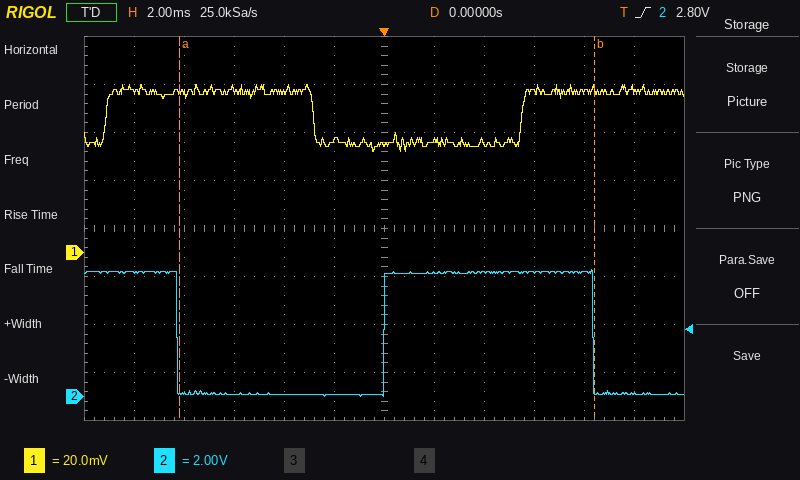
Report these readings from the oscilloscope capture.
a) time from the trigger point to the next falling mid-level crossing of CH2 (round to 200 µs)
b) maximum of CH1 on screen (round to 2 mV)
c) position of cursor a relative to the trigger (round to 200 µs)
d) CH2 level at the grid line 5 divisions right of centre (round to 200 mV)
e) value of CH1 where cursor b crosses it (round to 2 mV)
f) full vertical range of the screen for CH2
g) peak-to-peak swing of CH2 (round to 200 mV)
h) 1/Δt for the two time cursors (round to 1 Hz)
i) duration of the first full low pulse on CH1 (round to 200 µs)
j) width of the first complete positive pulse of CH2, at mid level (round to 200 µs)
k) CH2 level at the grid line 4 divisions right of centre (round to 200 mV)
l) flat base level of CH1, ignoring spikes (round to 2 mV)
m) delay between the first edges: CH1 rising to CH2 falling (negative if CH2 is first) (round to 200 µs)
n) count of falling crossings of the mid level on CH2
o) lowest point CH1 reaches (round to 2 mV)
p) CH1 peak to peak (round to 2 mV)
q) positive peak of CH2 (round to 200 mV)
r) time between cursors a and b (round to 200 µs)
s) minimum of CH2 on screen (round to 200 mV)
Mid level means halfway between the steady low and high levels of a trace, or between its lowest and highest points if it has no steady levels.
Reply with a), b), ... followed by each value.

a) 8.4 ms
b) 70 mV
c) -8.2 ms
d) 200 mV
e) 68 mV
f) 16 V
g) 5.2 V
h) 60 Hz
i) 8.4 ms
j) 8.4 ms
k) 5.2 V
l) 46 mV
m) +2.8 ms
n) 2
o) 42 mV
p) 28 mV
q) 5.2 V
r) 16.6 ms
s) 0.0 V
